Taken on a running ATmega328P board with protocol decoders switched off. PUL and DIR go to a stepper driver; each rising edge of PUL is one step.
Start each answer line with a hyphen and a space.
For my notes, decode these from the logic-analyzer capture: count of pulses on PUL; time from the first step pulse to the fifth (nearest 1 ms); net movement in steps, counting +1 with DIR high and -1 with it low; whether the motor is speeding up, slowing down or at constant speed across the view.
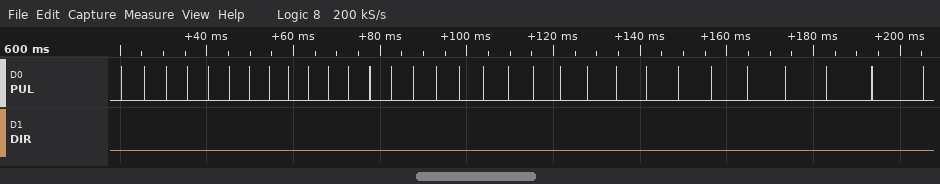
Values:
- 31
- 20 ms
- -31
- slowing down
